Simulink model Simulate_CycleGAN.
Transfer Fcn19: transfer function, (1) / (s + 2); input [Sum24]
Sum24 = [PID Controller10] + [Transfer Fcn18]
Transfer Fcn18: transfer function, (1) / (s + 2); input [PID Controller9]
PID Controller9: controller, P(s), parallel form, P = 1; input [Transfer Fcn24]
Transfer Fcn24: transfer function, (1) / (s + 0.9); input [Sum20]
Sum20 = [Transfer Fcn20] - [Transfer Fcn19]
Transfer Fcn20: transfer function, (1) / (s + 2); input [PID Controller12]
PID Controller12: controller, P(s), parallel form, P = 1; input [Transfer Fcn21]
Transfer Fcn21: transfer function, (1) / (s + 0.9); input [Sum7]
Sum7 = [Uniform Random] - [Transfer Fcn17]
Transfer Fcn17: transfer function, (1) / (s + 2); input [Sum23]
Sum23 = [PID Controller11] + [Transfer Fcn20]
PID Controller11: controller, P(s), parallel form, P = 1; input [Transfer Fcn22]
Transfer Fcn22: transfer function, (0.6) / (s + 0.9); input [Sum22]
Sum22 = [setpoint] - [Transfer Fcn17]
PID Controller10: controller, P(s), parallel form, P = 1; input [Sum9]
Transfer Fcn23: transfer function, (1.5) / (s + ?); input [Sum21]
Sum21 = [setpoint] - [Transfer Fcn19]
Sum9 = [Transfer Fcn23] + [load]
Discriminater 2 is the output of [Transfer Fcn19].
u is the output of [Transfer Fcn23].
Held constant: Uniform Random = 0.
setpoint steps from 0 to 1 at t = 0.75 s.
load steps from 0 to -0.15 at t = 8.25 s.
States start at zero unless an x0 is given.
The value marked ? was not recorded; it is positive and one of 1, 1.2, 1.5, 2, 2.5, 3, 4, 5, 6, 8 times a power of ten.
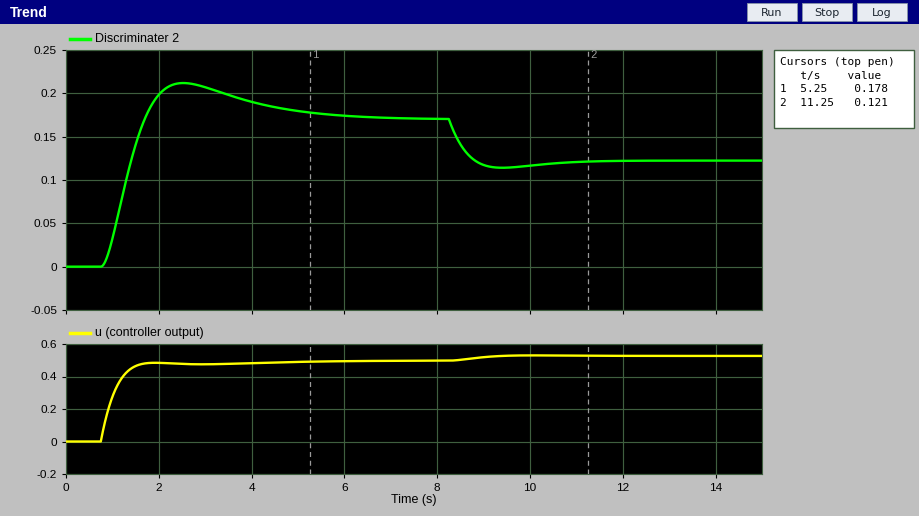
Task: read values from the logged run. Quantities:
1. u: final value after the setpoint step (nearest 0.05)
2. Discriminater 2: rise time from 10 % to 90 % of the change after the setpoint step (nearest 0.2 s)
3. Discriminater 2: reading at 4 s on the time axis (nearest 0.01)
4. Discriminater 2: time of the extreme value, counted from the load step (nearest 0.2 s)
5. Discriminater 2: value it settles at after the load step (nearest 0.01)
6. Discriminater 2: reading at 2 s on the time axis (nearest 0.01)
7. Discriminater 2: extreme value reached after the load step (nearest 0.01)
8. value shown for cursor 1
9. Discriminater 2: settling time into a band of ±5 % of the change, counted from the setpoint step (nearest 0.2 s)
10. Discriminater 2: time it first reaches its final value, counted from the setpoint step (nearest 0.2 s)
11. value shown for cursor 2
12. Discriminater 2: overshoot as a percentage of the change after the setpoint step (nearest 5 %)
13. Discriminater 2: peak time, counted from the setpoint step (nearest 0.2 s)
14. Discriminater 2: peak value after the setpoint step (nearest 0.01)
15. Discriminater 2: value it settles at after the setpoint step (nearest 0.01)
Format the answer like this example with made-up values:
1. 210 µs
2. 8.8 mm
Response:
1. 0.50
2. 0.6 s
3. 0.19
4. 1.2 s
5. 0.12
6. 0.20
7. 0.11
8. 0.178
9. 4.4 s
10. 1.0 s
11. 0.121
12. 25 %
13. 1.8 s
14. 0.21
15. 0.17
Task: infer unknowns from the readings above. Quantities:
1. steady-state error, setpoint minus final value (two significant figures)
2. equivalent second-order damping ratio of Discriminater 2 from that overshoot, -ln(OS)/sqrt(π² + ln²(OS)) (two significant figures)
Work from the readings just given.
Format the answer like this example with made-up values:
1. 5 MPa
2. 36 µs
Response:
1. 0.83
2. 0.40
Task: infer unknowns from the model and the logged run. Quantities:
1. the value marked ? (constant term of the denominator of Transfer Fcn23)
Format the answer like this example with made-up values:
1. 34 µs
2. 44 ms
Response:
1. 2.5
